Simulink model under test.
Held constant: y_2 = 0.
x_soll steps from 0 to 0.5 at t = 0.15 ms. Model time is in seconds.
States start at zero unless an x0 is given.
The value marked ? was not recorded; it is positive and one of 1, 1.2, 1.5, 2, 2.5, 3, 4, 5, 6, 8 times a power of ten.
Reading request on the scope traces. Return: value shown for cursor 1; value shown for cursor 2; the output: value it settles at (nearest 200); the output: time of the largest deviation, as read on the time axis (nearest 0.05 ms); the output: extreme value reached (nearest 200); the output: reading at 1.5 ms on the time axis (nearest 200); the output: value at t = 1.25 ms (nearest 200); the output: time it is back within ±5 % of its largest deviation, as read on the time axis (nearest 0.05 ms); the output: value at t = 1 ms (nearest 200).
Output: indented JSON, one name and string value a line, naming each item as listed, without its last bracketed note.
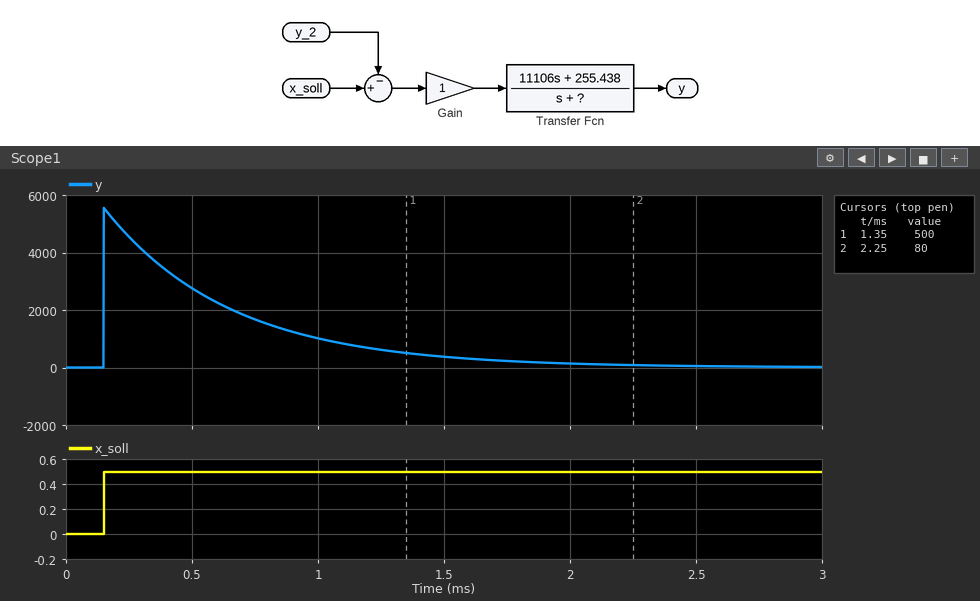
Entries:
{
  "value shown for cursor 1": "500",
  "value shown for cursor 2": "80",
  "the output: value it settles at": "0",
  "the output: time of the largest deviation, as read on the time axis": "0.15 ms",
  "the output: extreme value reached": "5600",
  "the output: reading at 1.5 ms on the time axis": "400",
  "the output: value at t = 1.25 ms": "600",
  "the output: time it is back within ±5 % of its largest deviation, as read on the time axis": "1.65 ms",
  "the output: value at t = 1 ms": "1000"
}
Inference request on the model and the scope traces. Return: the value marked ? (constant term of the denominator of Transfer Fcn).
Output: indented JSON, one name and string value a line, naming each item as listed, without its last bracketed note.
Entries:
{
  "the value marked ?": "2000"
}
